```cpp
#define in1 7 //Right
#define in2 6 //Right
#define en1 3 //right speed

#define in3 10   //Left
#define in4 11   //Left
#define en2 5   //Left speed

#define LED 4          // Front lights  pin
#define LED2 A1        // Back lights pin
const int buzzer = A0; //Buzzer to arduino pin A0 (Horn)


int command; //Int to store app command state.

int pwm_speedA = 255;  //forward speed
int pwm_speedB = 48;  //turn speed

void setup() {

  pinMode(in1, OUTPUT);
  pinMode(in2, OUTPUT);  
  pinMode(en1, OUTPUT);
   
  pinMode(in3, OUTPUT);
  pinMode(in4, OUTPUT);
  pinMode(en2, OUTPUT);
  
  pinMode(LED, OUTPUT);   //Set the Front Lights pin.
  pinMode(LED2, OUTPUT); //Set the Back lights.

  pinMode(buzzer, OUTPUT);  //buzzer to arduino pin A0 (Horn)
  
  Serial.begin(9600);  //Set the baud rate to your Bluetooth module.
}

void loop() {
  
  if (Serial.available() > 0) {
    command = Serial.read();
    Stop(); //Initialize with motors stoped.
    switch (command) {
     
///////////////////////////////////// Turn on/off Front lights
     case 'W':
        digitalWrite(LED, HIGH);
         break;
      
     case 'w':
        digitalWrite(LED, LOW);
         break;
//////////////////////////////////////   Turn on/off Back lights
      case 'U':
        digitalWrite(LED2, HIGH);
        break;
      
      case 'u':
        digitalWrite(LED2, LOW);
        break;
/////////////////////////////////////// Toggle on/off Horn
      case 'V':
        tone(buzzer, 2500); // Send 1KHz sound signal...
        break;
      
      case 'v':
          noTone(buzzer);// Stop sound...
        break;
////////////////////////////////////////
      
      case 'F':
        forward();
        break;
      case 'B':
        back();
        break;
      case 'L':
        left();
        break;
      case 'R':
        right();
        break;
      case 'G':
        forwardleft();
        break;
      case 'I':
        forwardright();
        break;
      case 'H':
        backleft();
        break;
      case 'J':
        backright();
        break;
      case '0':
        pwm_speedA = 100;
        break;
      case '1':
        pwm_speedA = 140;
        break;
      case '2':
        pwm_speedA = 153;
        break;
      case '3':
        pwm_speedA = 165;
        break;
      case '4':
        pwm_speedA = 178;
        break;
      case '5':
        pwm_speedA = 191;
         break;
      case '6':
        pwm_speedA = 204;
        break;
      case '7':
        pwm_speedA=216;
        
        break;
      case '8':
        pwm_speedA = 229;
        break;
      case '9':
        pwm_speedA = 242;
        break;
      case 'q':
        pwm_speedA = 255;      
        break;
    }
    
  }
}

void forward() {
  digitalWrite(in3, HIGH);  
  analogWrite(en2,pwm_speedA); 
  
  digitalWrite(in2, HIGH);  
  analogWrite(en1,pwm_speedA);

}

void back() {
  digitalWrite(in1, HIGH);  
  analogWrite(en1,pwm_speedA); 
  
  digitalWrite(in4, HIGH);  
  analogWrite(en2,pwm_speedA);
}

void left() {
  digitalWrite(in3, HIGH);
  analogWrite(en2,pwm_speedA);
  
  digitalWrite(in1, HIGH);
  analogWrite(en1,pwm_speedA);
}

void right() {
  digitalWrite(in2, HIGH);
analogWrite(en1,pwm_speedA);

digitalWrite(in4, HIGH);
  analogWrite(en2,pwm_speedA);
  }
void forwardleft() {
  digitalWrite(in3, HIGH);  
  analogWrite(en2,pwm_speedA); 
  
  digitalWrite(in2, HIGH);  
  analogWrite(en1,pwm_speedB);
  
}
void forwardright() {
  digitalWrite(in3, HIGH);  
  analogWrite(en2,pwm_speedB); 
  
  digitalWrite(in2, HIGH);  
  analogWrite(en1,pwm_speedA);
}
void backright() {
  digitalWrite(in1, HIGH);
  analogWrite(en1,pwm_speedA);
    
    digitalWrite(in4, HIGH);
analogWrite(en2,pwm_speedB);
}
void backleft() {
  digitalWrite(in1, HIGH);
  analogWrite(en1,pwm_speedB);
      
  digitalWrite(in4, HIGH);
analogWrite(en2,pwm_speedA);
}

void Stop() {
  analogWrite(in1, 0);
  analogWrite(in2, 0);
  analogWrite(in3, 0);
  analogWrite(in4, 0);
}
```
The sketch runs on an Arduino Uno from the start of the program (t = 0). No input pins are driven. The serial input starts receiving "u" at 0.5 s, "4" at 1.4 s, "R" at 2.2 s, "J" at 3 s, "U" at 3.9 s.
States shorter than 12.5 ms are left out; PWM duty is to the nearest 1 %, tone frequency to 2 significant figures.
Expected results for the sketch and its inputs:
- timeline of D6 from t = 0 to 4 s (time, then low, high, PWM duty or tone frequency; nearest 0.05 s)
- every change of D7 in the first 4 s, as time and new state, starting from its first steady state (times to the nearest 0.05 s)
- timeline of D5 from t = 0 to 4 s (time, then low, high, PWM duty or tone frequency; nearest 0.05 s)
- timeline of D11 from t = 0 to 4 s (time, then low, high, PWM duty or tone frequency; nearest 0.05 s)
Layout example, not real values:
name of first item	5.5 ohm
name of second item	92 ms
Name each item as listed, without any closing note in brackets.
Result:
timeline of D6 from t = 0 to 4 s	0 s low; 2.2 s high; 3 s low
every change of D7 in the first 4 s, as time and new state, starting from its first steady state	0 s low; 3 s high; 3.9 s low
timeline of D5 from t = 0 to 4 s	0 s low; 2.2 s PWM 70 %; 3 s PWM 19 %
timeline of D11 from t = 0 to 4 s	0 s low; 2.2 s high; 3.9 s low
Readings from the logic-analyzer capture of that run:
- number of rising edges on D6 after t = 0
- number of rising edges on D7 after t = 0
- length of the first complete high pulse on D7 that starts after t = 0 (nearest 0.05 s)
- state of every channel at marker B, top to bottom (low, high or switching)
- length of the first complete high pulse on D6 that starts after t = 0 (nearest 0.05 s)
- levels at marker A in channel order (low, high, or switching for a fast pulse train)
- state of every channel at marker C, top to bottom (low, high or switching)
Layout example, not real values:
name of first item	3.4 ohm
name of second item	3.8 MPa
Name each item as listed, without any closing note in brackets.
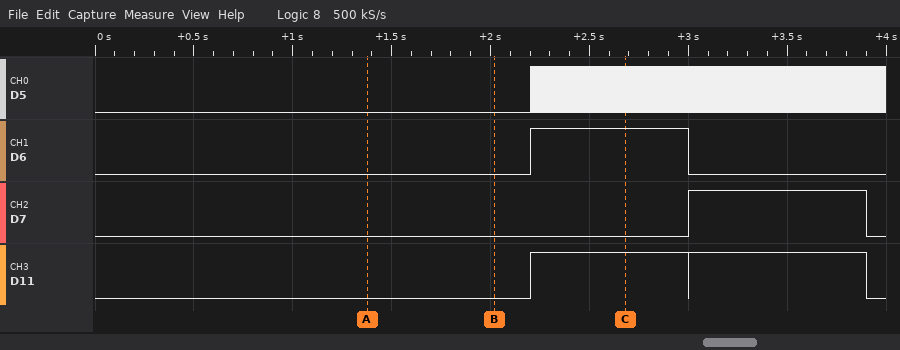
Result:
number of rising edges on D6 after t = 0	1
number of rising edges on D7 after t = 0	1
length of the first complete high pulse on D7 that starts after t = 0	0.90 s
state of every channel at marker B, top to bottom	D5 low, D6 low, D7 low, D11 low
length of the first complete high pulse on D6 that starts after t = 0	0.80 s
levels at marker A in channel order	D5 low, D6 low, D7 low, D11 low
state of every channel at marker C, top to bottom	D5 switching, D6 high, D7 low, D11 high
